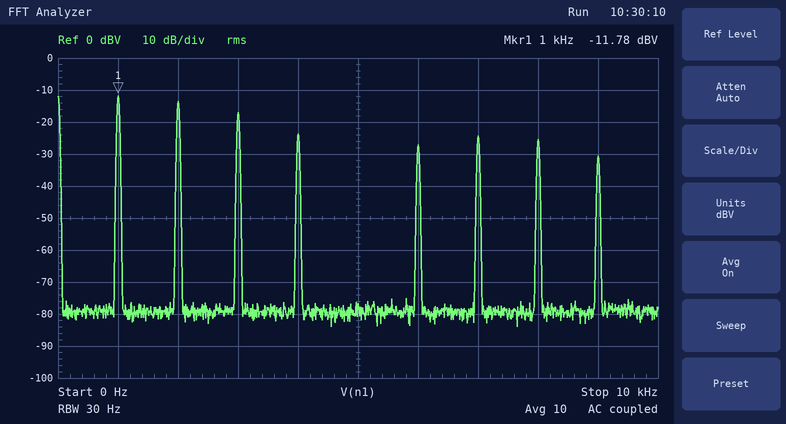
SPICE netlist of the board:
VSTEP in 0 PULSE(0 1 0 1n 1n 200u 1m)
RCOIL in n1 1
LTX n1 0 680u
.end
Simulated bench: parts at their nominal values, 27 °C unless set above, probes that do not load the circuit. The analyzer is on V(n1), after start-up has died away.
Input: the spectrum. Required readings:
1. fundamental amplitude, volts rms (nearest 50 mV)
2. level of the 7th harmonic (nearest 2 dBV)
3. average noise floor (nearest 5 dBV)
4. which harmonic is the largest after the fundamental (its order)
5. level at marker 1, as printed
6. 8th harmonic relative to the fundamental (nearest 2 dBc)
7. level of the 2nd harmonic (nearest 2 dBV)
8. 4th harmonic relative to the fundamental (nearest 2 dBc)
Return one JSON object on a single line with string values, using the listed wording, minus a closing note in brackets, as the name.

{"fundamental amplitude, volts rms": "250 mV", "level of the 7th harmonic": "-24 dBV", "average noise floor": "-80 dBV", "which harmonic is the largest after the fundamental": "2", "level at marker 1, as printed": "-11.78 dBV", "8th harmonic relative to the fundamental": "-14 dBc", "level of the 2nd harmonic": "-14 dBV", "4th harmonic relative to the fundamental": "-12 dBc"}
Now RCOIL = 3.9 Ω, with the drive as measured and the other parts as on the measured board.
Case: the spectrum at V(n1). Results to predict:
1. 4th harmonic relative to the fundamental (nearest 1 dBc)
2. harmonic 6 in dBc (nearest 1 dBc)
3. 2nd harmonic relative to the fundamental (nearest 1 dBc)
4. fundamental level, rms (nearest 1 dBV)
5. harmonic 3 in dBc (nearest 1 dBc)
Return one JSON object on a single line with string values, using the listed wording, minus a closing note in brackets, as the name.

{"4th harmonic relative to the fundamental": "-10 dBc", "harmonic 6 in dBc": "-13 dBc", "2nd harmonic relative to the fundamental": "0 dBc", "fundamental level, rms": "-14 dBV", "harmonic 3 in dBc": "-3 dBc"}
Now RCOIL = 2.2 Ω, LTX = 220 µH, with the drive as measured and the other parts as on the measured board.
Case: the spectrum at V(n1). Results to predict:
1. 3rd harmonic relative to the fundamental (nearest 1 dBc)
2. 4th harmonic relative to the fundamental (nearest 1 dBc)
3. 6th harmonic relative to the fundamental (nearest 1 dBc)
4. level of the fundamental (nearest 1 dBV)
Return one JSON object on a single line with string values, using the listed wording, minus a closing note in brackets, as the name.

{"3rd harmonic relative to the fundamental": "-1 dBc", "4th harmonic relative to the fundamental": "-7 dBc", "6th harmonic relative to the fundamental": "-10 dBc", "level of the fundamental": "-17 dBV"}
